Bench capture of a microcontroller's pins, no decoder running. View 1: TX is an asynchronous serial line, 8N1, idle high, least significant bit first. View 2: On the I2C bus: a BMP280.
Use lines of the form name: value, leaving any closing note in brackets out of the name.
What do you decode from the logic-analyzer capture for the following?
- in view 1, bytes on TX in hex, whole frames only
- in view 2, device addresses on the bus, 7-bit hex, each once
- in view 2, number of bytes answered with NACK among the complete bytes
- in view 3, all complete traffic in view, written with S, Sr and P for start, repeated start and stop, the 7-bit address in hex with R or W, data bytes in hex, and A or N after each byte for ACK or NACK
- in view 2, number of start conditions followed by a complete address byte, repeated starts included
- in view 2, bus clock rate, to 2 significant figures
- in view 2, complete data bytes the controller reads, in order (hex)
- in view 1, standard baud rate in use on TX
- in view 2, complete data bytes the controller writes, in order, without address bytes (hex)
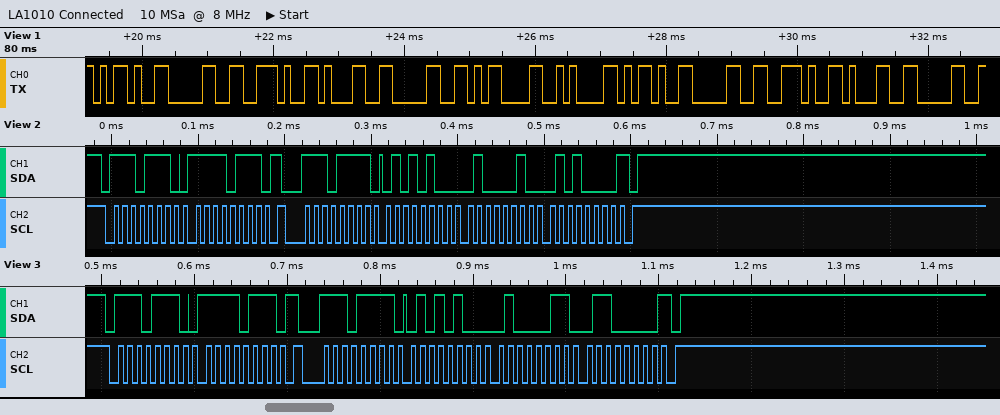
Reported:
in view 1, bytes on TX in hex, whole frames only: 2D 30 2E 31 30 0D 0A 2D 30 2E 31 30
in view 2, device addresses on the bus, 7-bit hex, each once: 0x77
in view 2, number of bytes answered with NACK among the complete bytes: 1
in view 3, all complete traffic in view, written with S, Sr and P for start, repeated start and stop, the 7-bit address in hex with R or W, data bytes in hex, and A or N after each byte for ACK or NACK: S 77W A F7 A Sr 77R A 54 A 43 A 60 N P
in view 2, number of start conditions followed by a complete address byte, repeated starts included: 2
in view 2, bus clock rate, to 2 significant figures: 100 kHz
in view 2, complete data bytes the controller reads, in order: 54 42 50
in view 1, standard baud rate in use on TX: 9600 baud
in view 2, complete data bytes the controller writes, in order, without address bytes: F7
